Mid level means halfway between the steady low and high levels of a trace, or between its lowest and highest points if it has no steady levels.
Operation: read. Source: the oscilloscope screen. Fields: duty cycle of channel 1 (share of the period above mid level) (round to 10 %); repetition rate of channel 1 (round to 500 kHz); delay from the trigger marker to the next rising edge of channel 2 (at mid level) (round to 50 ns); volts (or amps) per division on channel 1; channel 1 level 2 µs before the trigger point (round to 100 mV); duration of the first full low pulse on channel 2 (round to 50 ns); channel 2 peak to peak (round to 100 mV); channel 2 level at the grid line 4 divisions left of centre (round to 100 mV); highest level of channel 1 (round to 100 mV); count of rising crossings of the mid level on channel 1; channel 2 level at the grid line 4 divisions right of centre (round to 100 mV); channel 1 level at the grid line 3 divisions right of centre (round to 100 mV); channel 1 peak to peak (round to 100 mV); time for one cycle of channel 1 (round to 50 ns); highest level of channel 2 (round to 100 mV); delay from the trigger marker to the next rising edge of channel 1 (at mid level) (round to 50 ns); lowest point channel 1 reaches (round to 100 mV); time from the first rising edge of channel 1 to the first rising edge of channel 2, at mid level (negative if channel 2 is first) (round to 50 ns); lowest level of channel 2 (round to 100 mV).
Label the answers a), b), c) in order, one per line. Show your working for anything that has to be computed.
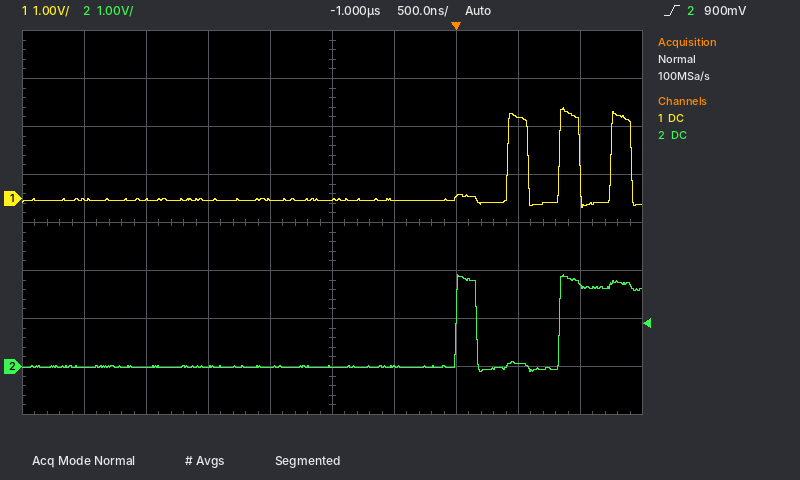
a) 40 %
b) 1 / 400 ns ≈ 2.5 MHz
c) 850 ns
d) 1 V
e) 0.0 V
f) 650 ns
g) 1.9 V − (-100 mV) = 2.0 V
h) 0.0 V
i) 1.9 V
j) 3
k) 1.7 V
l) 1.7 V
m) 1.9 V − (-200 mV) = 2.1 V
n) 400 ns
o) 1.9 V
p) 400 ns
q) -200 mV
r) -400 ns
s) -100 mV
